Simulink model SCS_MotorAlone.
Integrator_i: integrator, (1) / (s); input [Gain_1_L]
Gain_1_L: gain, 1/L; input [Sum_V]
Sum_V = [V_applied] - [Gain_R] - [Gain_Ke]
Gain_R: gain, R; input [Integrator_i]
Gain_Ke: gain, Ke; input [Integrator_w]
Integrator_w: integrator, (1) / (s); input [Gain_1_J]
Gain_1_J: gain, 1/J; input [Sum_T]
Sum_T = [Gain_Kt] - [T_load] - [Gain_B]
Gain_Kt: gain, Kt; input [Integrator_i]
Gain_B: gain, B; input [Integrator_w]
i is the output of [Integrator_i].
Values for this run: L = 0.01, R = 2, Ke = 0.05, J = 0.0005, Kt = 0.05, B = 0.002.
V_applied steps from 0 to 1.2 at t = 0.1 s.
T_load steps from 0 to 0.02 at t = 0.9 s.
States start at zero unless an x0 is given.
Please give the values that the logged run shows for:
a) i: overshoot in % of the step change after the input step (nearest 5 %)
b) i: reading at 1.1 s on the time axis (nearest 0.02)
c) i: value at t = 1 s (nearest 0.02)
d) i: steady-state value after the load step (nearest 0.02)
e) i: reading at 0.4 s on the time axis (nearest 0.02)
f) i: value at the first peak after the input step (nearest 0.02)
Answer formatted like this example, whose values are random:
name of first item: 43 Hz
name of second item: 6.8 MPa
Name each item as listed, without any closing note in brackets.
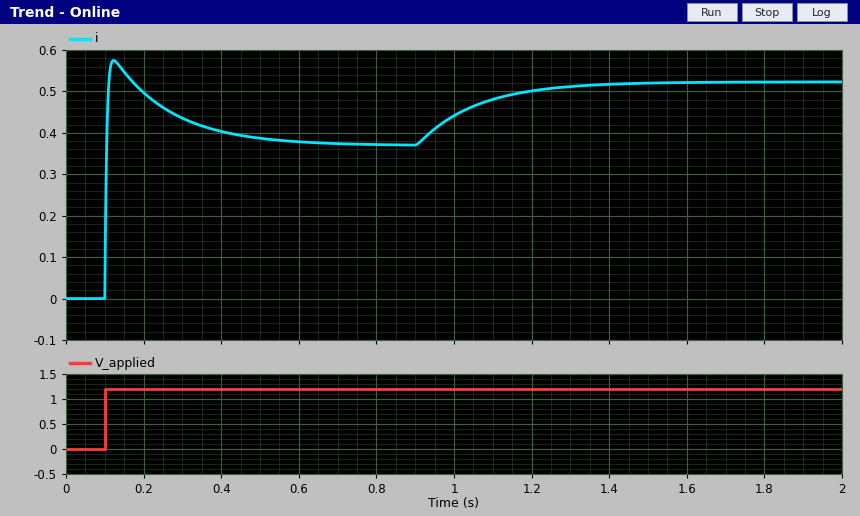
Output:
i: overshoot in % of the step change after the input step: 55 %
i: reading at 1.1 s on the time axis: 0.48
i: value at t = 1 s: 0.44
i: steady-state value after the load step: 0.52
i: reading at 0.4 s on the time axis: 0.40
i: value at the first peak after the input step: 0.58
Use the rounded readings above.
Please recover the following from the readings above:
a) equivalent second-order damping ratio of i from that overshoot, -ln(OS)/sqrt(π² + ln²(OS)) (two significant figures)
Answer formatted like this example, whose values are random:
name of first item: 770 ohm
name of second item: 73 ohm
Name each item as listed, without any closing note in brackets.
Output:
equivalent second-order damping ratio of i from that overshoot, -ln(OS)/sqrt(π² + ln²(OS)): 0.19
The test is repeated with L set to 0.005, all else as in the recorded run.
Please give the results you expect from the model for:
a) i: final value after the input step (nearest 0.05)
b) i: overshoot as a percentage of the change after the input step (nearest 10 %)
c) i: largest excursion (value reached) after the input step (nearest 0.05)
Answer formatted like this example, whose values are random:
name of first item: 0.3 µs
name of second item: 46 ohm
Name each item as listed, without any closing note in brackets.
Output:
i: final value after the input step: 0.35
i: overshoot as a percentage of the change after the input step: 60 %
i: largest excursion (value reached) after the input step: 0.60
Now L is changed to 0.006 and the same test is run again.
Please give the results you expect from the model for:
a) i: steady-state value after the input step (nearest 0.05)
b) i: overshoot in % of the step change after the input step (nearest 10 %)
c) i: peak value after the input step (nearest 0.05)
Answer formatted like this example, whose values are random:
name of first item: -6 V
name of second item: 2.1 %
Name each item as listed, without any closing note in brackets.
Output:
i: steady-state value after the input step: 0.35
i: overshoot in % of the step change after the input step: 60 %
i: peak value after the input step: 0.60
